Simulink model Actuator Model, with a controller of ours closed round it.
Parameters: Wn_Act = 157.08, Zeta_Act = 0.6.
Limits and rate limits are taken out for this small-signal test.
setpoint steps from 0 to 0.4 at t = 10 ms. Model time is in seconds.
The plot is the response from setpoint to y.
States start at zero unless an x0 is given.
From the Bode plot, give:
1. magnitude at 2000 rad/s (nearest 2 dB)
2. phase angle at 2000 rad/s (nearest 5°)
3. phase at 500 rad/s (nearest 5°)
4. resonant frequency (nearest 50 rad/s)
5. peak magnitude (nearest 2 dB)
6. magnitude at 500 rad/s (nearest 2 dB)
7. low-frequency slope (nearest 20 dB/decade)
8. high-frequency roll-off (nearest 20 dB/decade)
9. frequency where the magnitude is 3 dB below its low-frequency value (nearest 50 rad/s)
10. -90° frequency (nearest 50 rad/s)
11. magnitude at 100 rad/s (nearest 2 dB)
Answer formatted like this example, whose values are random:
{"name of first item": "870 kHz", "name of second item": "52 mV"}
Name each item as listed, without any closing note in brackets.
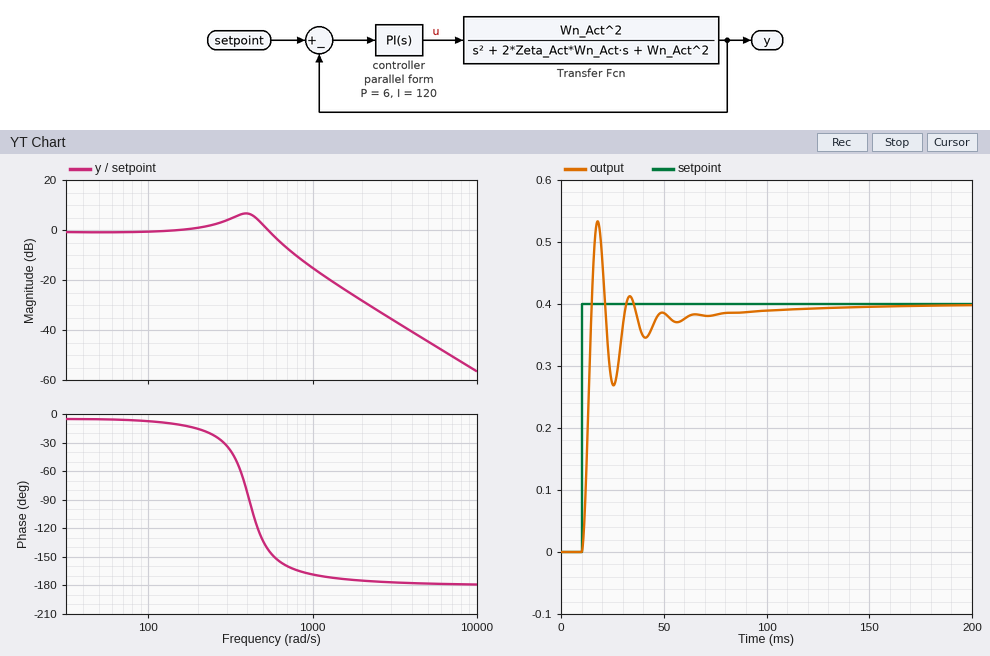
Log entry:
{"magnitude at 2000 rad/s": "-28 dB", "phase angle at 2000 rad/s": "-175°", "phase at 500 rad/s": "-135°", "resonant frequency": "400 rad/s", "peak magnitude": "6 dB", "magnitude at 500 rad/s": "2 dB", "low-frequency slope": "0 dB/decade", "high-frequency roll-off": "-40 dB/decade", "frequency where the magnitude is 3 dB below its low-frequency value": "600 rad/s", "-90° frequency": "400 rad/s", "magnitude at 100 rad/s": "0 dB"}
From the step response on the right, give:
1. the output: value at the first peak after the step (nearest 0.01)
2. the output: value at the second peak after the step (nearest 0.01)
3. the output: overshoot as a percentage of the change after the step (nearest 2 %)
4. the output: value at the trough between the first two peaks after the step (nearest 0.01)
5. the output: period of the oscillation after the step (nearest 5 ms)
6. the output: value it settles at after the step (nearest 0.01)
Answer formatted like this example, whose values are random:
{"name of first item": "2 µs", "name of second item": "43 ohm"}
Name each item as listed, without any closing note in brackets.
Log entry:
{"the output: value at the first peak after the step": "0.53", "the output: value at the second peak after the step": "0.41", "the output: overshoot as a percentage of the change after the step": "34 %", "the output: value at the trough between the first two peaks after the step": "0.27", "the output: period of the oscillation after the step": "15 ms", "the output: value it settles at after the step": "0.40"}
